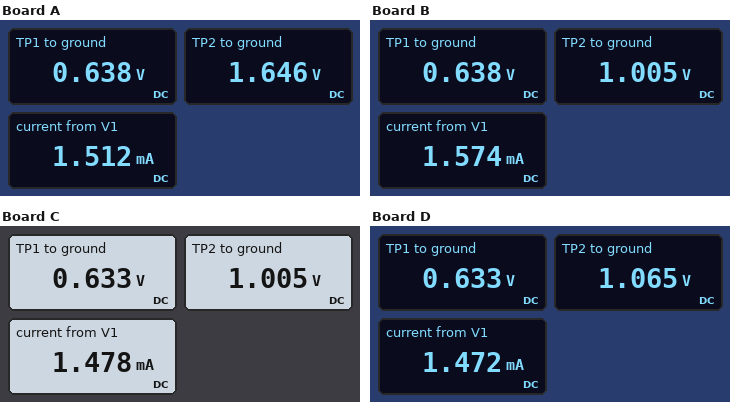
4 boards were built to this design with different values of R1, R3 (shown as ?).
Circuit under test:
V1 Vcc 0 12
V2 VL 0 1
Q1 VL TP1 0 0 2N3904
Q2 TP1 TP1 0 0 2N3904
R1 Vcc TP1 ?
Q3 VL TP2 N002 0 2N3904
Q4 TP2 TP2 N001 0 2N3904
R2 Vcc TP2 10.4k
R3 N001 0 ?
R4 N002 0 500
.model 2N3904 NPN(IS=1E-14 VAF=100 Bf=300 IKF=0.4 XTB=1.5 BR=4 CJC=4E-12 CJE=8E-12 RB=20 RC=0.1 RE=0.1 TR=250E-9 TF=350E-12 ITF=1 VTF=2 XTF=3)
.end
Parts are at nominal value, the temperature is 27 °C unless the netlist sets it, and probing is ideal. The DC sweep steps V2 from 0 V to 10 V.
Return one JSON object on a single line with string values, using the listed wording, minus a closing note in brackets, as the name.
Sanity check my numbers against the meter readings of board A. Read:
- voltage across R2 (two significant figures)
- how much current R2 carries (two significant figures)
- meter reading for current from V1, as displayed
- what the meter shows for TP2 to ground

{"voltage across R2": "10 V", "how much current R2 carries": "1.0 mA", "meter reading for current from V1, as displayed": "1.512 mA", "what the meter shows for TP2 to ground": "1.646 V"}
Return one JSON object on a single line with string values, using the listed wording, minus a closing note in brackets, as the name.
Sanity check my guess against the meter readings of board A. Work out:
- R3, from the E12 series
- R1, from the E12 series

{"R3, from the E12 series": "1.2 kΩ", "R1, from the E12 series": "22 kΩ"}
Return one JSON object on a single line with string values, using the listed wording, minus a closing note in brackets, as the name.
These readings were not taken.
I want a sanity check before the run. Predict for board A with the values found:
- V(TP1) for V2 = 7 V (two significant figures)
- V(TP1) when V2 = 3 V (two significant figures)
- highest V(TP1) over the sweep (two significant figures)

{"V(TP1) for V2 = 7 V": "640 mV", "V(TP1) when V2 = 3 V": "640 mV", "highest V(TP1) over the sweep": "640 mV"}
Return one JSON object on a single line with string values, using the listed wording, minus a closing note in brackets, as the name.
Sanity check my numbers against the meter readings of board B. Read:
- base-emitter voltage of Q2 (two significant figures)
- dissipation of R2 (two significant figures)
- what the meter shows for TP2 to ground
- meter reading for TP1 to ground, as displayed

{"base-emitter voltage of Q2": "640 mV", "dissipation of R2": "12 mW", "what the meter shows for TP2 to ground": "1.005 V", "meter reading for TP1 to ground, as displayed": "0.638 V"}
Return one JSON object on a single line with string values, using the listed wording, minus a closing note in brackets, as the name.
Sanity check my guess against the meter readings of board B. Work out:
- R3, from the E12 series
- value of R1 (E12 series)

{"R3, from the E12 series": "330 Ω", "value of R1": "22 kΩ"}
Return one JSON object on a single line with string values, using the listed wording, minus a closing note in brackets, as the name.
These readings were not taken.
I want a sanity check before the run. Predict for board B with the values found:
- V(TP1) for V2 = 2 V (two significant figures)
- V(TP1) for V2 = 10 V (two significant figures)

{"V(TP1) for V2 = 2 V": "640 mV", "V(TP1) for V2 = 10 V": "640 mV"}
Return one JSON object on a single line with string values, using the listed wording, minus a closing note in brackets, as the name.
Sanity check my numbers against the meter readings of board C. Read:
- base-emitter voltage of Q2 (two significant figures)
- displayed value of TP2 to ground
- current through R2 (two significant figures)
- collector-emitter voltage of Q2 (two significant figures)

{"base-emitter voltage of Q2": "630 mV", "displayed value of TP2 to ground": "1.005 V", "current through R2": "1.1 mA", "collector-emitter voltage of Q2": "630 mV"}
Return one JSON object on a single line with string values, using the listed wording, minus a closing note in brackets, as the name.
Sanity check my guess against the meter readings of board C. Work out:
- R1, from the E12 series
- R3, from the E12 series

{"R1, from the E12 series": "27 kΩ", "R3, from the E12 series": "330 Ω"}
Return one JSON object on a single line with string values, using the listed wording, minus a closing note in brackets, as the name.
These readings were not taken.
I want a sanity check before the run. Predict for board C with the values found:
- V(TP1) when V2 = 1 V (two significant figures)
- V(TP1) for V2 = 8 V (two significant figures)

{"V(TP1) when V2 = 1 V": "630 mV", "V(TP1) for V2 = 8 V": "630 mV"}
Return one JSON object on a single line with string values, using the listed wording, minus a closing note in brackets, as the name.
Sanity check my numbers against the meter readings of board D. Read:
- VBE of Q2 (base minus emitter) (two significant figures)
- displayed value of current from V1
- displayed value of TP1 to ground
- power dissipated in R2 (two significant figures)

{"VBE of Q2 (base minus emitter)": "630 mV", "displayed value of current from V1": "1.472 mA", "displayed value of TP1 to ground": "0.633 V", "power dissipated in R2": "11 mW"}
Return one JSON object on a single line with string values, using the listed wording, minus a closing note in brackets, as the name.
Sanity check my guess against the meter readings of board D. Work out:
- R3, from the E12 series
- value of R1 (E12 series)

{"R3, from the E12 series": "390 Ω", "value of R1": "27 kΩ"}
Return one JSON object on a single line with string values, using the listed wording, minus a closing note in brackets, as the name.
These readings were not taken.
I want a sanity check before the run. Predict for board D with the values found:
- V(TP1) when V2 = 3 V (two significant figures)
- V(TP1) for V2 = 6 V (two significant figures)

{"V(TP1) when V2 = 3 V": "630 mV", "V(TP1) for V2 = 6 V": "630 mV"}
